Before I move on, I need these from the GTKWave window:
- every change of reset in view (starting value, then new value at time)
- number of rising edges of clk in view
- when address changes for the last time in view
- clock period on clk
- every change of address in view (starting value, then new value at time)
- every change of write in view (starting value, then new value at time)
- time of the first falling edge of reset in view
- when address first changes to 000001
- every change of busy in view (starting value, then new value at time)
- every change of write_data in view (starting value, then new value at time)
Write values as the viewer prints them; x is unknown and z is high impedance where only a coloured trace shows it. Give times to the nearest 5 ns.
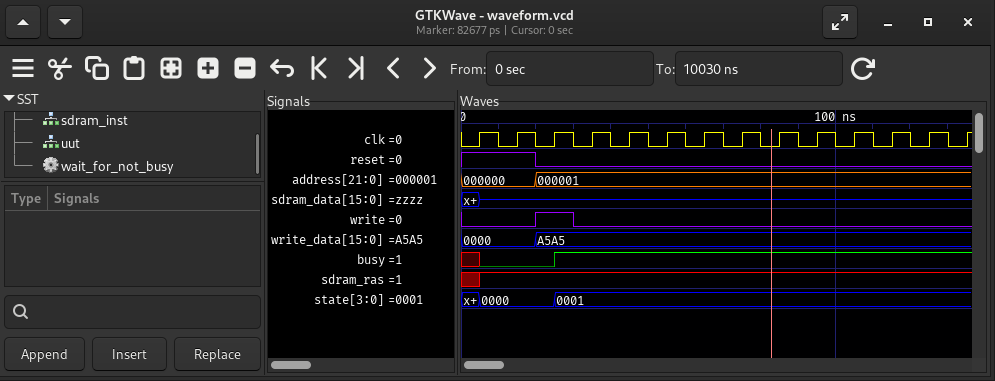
1, 0 at 20 ns
14
20 ns
10 ns
000000, 000001 at 20 ns
0, 1 at 20 ns, 0 at 30 ns
20 ns
20 ns
x, 0 at 5 ns, 1 at 25 ns
0000, A5A5 at 20 ns
